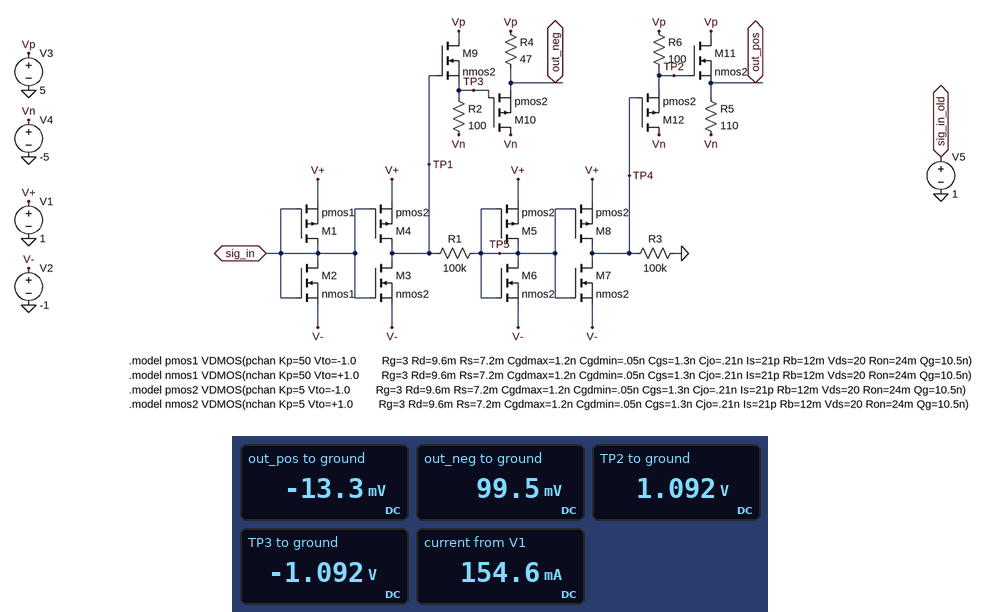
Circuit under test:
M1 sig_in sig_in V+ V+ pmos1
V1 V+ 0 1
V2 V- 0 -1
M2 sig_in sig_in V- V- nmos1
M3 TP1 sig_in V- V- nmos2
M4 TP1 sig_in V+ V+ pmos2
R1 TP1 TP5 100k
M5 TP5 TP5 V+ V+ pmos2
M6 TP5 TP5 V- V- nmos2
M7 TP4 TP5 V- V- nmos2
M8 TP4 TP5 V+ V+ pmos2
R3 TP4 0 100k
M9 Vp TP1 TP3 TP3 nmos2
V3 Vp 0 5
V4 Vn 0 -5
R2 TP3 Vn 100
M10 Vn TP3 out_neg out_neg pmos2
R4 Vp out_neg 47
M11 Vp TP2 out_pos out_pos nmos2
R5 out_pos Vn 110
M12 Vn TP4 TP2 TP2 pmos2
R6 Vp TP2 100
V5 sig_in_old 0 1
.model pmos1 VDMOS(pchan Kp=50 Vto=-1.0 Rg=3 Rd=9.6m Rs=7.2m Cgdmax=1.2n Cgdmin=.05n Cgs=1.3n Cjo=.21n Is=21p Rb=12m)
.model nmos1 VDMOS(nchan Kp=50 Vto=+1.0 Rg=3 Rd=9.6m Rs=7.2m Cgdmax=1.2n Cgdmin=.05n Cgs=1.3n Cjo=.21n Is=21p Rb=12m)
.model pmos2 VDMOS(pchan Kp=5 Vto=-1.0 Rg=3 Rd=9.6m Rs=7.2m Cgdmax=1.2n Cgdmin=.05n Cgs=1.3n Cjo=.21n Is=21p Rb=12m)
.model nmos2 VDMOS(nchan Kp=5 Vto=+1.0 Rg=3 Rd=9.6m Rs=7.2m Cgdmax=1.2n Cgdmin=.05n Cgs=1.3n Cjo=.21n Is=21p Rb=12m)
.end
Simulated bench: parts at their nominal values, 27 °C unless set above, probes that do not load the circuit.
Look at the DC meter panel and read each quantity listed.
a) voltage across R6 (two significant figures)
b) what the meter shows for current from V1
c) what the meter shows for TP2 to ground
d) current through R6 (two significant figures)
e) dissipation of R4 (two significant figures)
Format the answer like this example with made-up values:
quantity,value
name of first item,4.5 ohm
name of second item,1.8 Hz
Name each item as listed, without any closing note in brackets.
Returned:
quantity,value
voltage across R6,3.9 V
what the meter shows for current from V1,154.6 mA
what the meter shows for TP2 to ground,1.092 V
current through R6,39 mA
dissipation of R4,510 mW
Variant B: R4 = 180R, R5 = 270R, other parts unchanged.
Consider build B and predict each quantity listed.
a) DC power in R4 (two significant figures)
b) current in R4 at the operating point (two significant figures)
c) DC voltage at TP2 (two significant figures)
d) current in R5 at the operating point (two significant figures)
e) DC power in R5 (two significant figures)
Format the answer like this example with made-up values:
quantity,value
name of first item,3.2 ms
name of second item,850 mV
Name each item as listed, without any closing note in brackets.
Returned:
quantity,value
DC power in R4,140 mW
current in R4 at the operating point,28 mA
DC voltage at TP2,1.1 V
current in R5 at the operating point,19 mA
DC power in R5,95 mW
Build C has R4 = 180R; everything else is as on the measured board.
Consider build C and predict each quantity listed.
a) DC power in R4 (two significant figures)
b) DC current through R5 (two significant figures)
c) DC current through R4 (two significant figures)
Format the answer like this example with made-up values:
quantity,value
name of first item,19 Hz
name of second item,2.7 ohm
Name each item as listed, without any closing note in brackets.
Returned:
quantity,value
DC power in R4,140 mW
DC current through R5,45 mA
DC current through R4,28 mA
